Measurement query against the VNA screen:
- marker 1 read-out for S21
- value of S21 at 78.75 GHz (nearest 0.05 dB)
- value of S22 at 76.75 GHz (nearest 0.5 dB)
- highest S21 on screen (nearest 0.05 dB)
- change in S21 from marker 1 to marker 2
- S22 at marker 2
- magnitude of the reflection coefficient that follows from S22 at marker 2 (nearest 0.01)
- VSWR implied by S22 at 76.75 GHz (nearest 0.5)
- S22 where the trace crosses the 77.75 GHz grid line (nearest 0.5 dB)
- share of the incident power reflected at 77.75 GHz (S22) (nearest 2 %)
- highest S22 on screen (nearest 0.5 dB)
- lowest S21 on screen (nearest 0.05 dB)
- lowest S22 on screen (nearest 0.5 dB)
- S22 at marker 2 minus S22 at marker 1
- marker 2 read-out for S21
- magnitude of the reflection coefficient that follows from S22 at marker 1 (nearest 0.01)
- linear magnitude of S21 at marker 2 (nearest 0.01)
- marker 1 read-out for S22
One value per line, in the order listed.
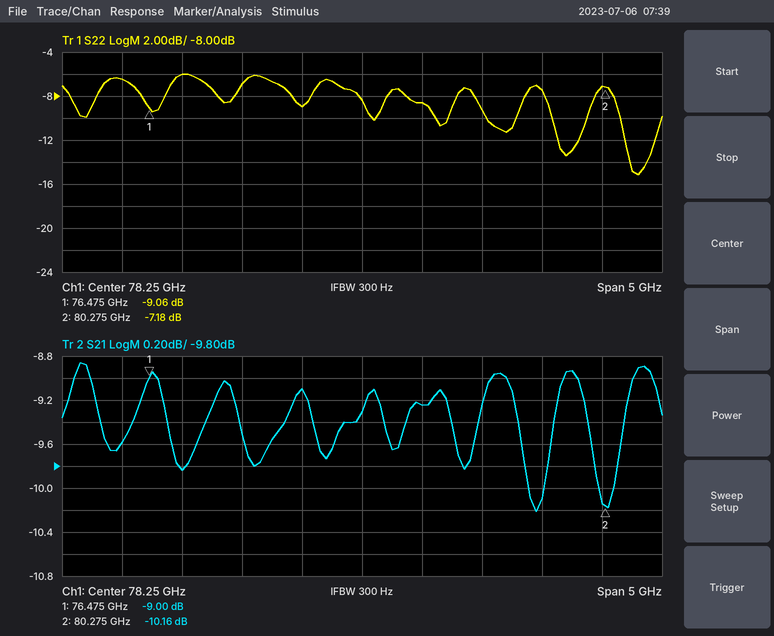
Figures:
-9.00 dB
-9.25 dB
-6.0 dB
-8.85 dB
-1.16 dB
-7.18 dB
0.44
3.0
-9.0 dB
12 %
-6.0 dB
-10.20 dB
-15.0 dB
1.88 dB
-10.16 dB
0.35
0.31
-9.06 dB
